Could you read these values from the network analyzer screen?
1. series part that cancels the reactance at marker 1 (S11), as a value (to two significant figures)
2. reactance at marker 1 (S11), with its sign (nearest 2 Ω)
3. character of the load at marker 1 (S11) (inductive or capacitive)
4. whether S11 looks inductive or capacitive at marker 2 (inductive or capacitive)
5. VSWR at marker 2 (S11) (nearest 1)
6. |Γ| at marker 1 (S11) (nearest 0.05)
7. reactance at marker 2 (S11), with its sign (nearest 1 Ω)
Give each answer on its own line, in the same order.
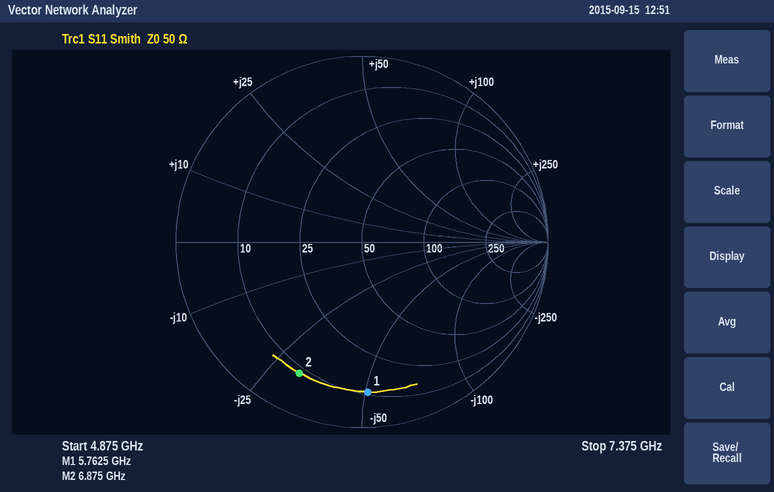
1.4 nH
-50 Ω
capacitive
capacitive
8
0.80
-31 Ω
